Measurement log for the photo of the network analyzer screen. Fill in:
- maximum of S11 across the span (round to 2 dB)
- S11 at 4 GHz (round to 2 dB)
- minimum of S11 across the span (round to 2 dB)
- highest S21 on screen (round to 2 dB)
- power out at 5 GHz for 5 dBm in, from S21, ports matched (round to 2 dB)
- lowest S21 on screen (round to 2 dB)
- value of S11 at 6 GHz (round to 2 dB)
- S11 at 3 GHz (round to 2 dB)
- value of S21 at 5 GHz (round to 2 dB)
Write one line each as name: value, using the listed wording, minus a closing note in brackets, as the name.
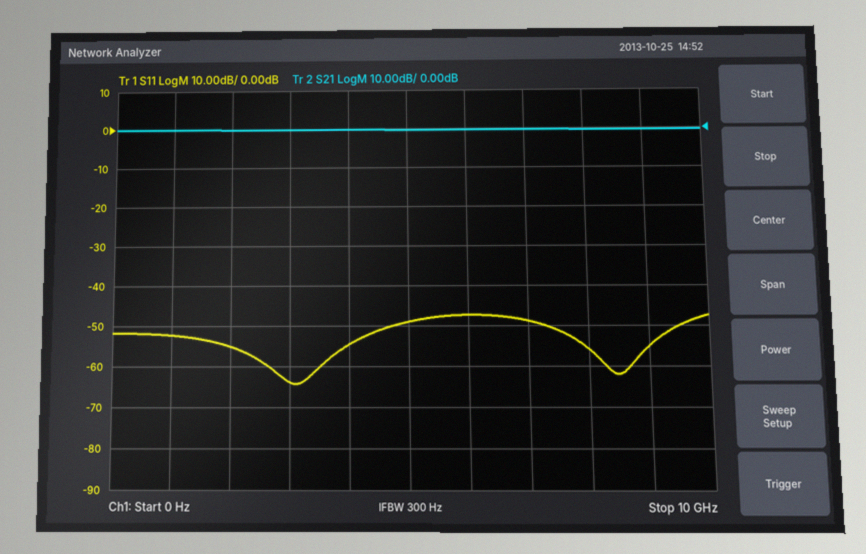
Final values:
maximum of S11 across the span: -48 dB
S11 at 4 GHz: -54 dB
minimum of S11 across the span: -64 dB
highest S21 on screen: 0 dB
power out at 5 GHz for 5 dBm in, from S21, ports matched: 4 dBm
lowest S21 on screen: 0 dB
value of S11 at 6 GHz: -48 dB
S11 at 3 GHz: -64 dB
value of S21 at 5 GHz: 0 dB
